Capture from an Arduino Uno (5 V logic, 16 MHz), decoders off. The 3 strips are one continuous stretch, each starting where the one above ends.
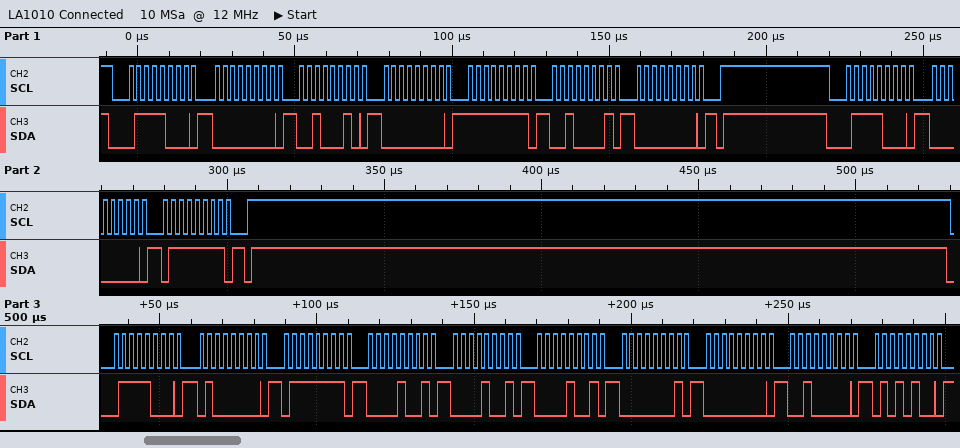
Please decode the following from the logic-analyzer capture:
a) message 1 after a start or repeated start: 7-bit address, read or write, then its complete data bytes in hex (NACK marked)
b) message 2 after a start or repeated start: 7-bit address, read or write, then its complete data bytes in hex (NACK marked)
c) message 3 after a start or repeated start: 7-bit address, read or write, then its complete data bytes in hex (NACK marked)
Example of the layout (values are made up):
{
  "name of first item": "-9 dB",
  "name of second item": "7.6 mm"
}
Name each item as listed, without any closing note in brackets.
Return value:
{
  "message 1 after a start or repeated start: 7-bit address, read or write, then its complete data bytes in hex": "0x3C write: 00 22 00 FF 21 00",
  "message 2 after a start or repeated start: 7-bit address, read or write, then its complete data bytes in hex": "0x3C write: 00 7F",
  "message 3 after a start or repeated start: 7-bit address, read or write, then its complete data bytes in hex": "0x3C write: 40 7F 09 09 09 01 00 20 54"
}
